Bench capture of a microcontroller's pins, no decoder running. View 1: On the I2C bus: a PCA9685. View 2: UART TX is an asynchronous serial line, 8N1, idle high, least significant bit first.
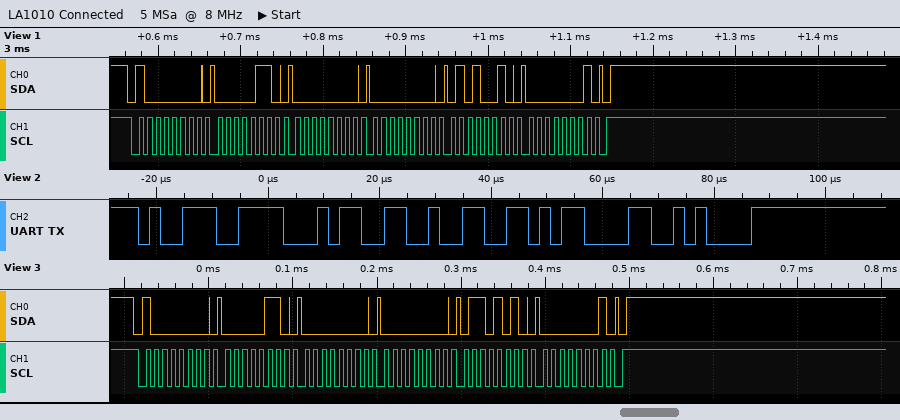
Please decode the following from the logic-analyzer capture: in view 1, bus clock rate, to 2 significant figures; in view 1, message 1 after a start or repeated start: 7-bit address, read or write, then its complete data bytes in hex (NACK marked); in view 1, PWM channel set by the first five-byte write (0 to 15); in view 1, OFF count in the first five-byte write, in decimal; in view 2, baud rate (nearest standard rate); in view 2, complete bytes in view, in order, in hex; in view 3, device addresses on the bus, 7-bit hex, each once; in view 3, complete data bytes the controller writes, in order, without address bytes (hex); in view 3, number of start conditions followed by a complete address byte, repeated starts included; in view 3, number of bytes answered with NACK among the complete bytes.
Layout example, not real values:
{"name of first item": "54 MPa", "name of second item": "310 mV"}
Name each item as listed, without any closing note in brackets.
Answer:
{"in view 1, bus clock rate, to 2 significant figures": "100 kHz", "in view 1, message 1 after a start or repeated start: 7-bit address, read or write, then its complete data bytes in hex": "0x40 write: 06 00 00 52 01", "in view 1, PWM channel set by the first five-byte write": "0", "in view 1, OFF count in the first five-byte write, in decimal": "338", "in view 2, baud rate": "500000 baud", "in view 2, complete bytes in view, in order, in hex": "0x39 0x34 0x32 0x0D 0x0A", "in view 3, device addresses on the bus, 7-bit hex, each once": "0x40", "in view 3, complete data bytes the controller writes, in order, without address bytes": "06 00 00 6A 01", "in view 3, number of start conditions followed by a complete address byte, repeated starts included": "1", "in view 3, number of bytes answered with NACK among the complete bytes": "0"}
